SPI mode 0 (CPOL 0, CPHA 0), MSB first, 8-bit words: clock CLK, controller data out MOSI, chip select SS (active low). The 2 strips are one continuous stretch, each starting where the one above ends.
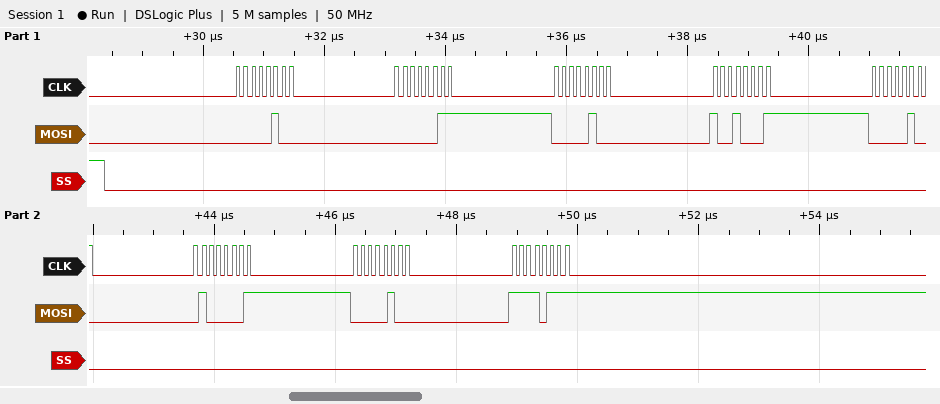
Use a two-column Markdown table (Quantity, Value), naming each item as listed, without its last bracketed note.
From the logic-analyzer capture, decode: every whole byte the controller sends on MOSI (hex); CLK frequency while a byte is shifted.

| Quantity | Value |
|---|---|
| every whole byte the controller sends on MOSI | 04 03 04 91 04 41 04 F7 |
| CLK frequency while a byte is shifted | 8 MHz |
